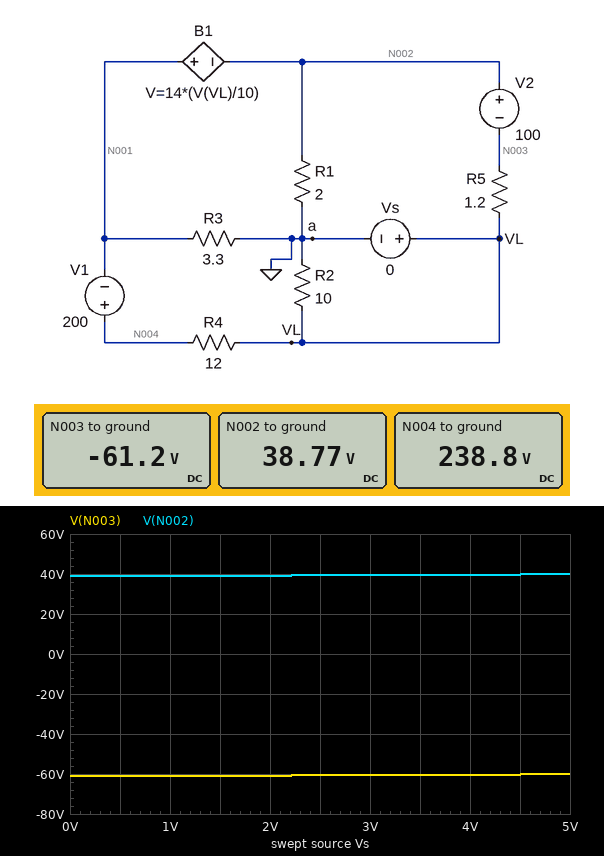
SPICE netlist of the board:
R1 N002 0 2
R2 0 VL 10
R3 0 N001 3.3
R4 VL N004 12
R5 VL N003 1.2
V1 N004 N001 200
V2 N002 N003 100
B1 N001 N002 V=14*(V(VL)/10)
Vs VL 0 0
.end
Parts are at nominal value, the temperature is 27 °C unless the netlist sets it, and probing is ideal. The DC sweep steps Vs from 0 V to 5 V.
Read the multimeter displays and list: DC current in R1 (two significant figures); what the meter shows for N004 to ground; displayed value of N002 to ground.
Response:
19 A
238.8 V
38.77 V
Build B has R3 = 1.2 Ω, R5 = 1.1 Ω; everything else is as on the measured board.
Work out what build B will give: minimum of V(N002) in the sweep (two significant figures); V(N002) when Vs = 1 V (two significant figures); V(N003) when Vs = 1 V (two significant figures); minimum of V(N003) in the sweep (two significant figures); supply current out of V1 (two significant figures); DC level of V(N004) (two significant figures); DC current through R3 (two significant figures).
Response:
31 V
32 V
-68 V
-69 V
19 A
230 V
27 A
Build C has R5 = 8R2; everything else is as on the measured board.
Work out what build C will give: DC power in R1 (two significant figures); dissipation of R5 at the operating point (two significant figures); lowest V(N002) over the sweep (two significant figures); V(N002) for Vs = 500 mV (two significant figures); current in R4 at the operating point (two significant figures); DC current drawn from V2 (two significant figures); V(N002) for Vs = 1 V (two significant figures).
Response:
9.8 W
1.3 kW
-6.1 V
-4.6 V
16 A
13 A
-4.8 V
